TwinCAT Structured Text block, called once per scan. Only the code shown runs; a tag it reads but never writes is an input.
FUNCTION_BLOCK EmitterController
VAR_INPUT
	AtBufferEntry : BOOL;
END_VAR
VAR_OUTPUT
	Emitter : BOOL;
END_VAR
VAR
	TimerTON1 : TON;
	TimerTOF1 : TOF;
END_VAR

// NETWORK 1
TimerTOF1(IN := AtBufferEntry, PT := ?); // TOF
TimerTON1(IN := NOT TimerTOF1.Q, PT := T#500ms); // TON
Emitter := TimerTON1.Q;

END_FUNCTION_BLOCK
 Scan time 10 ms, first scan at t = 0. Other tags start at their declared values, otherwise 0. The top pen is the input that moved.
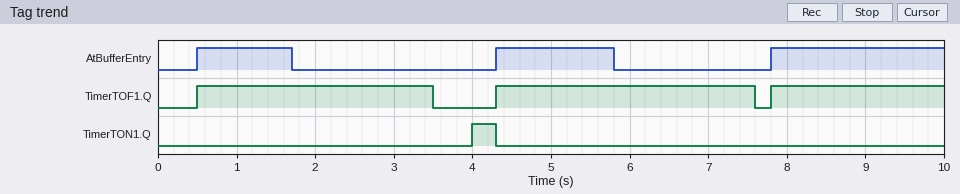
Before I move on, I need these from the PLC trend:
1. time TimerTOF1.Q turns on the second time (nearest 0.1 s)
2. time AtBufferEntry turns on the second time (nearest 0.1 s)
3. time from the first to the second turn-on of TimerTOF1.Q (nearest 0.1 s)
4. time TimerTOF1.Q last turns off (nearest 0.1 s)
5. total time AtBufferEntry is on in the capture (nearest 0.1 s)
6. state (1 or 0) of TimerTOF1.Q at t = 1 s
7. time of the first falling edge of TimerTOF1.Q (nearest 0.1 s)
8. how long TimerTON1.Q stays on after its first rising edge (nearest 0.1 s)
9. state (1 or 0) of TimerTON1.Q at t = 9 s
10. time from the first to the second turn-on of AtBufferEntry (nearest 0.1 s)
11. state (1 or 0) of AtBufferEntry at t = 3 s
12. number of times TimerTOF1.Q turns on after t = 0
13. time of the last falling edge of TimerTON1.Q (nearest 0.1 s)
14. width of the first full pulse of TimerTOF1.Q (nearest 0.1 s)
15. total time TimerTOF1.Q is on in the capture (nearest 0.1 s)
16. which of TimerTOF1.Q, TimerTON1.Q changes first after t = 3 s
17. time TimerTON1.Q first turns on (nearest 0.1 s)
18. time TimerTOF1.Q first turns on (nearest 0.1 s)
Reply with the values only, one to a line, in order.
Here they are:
4.3 s
4.3 s
3.8 s
7.6 s
4.9 s
1
3.5 s
0.3 s
0
3.8 s
0
3
4.3 s
3.0 s
8.5 s
TimerTOF1.Q
4.0 s
0.5 s
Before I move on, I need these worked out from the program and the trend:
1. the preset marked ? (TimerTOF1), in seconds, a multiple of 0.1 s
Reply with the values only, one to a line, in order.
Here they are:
1.8 s
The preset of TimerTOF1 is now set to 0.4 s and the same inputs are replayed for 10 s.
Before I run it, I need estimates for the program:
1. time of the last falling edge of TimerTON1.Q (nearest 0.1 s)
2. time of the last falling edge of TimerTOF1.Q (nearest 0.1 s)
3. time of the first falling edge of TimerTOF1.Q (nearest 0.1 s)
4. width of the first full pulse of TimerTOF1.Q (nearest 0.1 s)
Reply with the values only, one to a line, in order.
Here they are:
7.8 s
6.2 s
2.1 s
1.6 s
